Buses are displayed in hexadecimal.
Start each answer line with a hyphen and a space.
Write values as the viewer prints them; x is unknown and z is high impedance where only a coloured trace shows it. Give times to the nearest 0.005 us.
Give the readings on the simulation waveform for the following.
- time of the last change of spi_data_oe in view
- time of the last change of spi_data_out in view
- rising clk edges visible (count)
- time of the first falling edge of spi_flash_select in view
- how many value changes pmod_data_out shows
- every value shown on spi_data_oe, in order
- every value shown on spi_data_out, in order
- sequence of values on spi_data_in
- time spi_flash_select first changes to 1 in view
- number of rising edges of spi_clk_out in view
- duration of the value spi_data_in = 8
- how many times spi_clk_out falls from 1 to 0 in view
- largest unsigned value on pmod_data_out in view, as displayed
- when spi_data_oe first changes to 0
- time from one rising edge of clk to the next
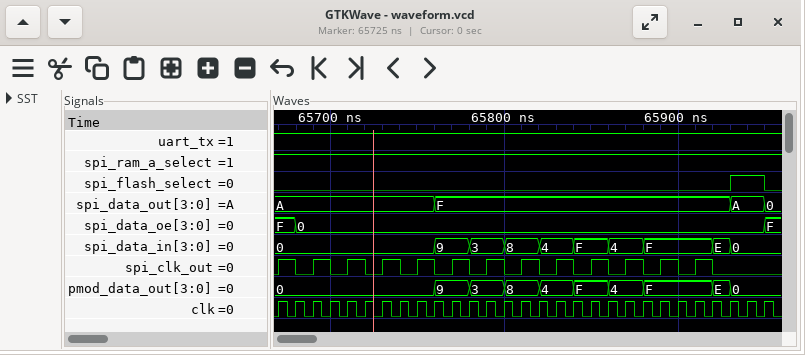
- 65.95 us
- 65.95 us
- 29
- 65.95 us
- 9
- F, 0, F
- A, F, A, 0
- 0, 9, 3, 8, 4, F, 4, F, E, 0
- 65.93 us
- 13
- 0.02 us
- 13
- F
- 65.68 us
- 0.01 us
